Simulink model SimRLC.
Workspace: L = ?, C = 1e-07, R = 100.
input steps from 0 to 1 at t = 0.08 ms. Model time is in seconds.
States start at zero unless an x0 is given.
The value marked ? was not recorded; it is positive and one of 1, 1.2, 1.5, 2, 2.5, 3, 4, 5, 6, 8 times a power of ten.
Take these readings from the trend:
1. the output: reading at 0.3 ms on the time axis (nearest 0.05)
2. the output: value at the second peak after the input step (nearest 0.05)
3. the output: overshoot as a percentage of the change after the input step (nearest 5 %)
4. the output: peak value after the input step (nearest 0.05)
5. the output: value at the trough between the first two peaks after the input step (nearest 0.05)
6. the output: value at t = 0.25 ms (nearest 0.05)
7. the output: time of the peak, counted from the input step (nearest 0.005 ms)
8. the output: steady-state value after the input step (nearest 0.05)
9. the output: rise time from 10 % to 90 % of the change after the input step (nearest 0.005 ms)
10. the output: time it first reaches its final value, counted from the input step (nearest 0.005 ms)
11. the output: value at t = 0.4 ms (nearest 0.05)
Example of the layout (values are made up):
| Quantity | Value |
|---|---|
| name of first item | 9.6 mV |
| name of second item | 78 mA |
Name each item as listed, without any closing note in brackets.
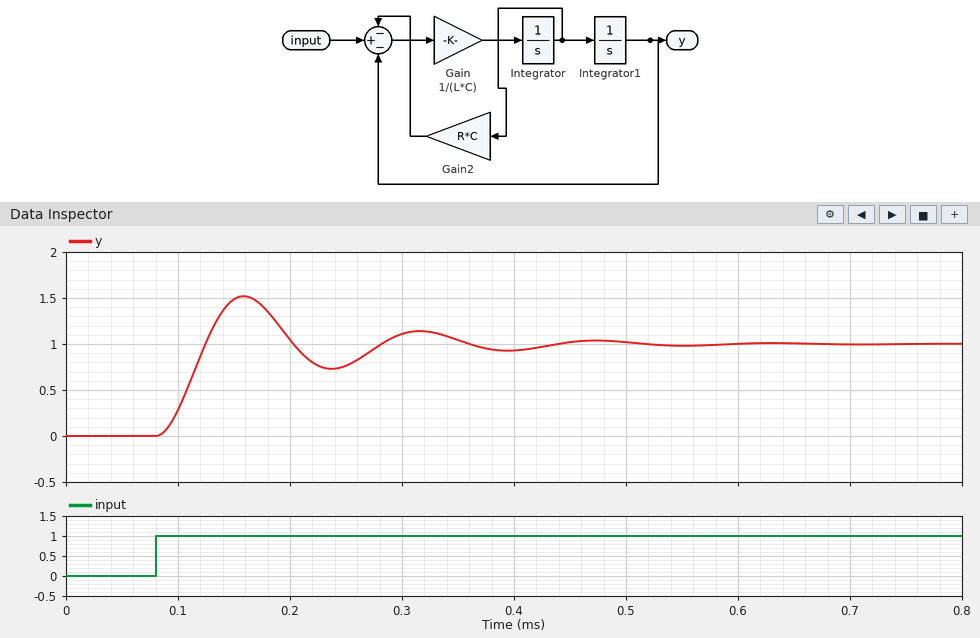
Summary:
| Quantity | Value |
|---|---|
| the output: reading at 0.3 ms on the time axis | 1.10 |
| the output: value at the second peak after the input step | 1.15 |
| the output: overshoot as a percentage of the change after the input step | 50 % |
| the output: peak value after the input step | 1.50 |
| the output: value at the trough between the first two peaks after the input step | 0.75 |
| the output: value at t = 0.25 ms | 0.75 |
| the output: time of the peak, counted from the input step | 0.080 ms |
| the output: steady-state value after the input step | 1.00 |
| the output: rise time from 10 % to 90 % of the change after the input step | 0.030 ms |
| the output: time it first reaches its final value, counted from the input step | 0.045 ms |
| the output: value at t = 0.4 ms | 0.95 |
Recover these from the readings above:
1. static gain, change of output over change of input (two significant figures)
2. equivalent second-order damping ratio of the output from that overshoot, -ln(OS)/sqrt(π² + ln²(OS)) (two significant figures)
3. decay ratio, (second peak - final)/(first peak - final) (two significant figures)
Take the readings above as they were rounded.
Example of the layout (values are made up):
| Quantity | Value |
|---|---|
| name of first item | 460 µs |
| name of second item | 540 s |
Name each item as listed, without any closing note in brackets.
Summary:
| Quantity | Value |
|---|---|
| static gain, change of output over change of input | 1.0 |
| equivalent second-order damping ratio of the output from that overshoot, -ln(OS)/sqrt(π² + ln²(OS)) | 0.22 |
| decay ratio, (second peak - final)/(first peak - final) | 0.30 |
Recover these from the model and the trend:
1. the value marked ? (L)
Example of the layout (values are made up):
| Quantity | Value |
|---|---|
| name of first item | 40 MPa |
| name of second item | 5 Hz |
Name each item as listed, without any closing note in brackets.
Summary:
| Quantity | Value |
|---|---|
| the value marked ? | 0.006 |
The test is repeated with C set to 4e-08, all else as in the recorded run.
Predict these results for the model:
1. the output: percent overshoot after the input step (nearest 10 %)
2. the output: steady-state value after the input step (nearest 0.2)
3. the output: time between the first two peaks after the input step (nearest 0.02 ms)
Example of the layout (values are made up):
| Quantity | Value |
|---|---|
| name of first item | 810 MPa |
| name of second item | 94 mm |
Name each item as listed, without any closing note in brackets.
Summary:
| Quantity | Value |
|---|---|
| the output: percent overshoot after the input step | 70 % |
| the output: steady-state value after the input step | 1.0 |
| the output: time between the first two peaks after the input step | 0.10 ms |
